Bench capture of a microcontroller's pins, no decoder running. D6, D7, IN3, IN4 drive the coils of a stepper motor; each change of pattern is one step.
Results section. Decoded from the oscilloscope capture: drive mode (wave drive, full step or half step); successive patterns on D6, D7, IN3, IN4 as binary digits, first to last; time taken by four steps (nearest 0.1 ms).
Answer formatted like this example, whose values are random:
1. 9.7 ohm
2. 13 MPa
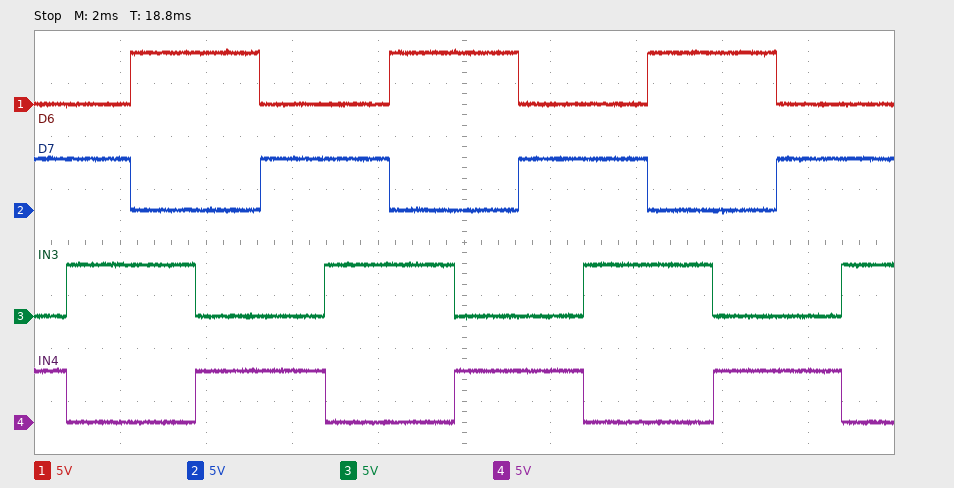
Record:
1. full step
2. 0101 0110 1010 1001 0101 0110 1010 1001 0101 0110 1010 1001 0101 0110
3. 6.0 ms
